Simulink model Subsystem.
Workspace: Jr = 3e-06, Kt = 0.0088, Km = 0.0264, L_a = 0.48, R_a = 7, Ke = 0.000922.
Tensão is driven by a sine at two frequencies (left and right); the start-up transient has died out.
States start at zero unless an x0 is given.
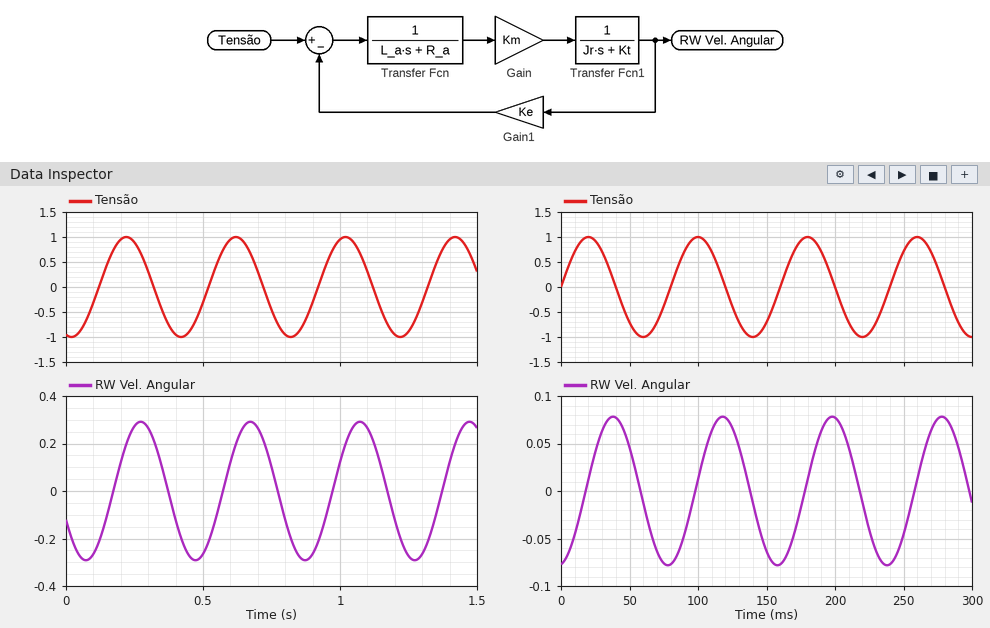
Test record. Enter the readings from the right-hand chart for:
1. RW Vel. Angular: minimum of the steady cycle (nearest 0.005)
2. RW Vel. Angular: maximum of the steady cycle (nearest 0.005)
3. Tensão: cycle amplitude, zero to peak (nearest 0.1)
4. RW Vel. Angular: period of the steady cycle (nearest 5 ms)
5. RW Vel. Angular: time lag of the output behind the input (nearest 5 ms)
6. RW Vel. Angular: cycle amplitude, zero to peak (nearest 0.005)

-0.080
0.080
1.0
80 ms
20 ms
0.080
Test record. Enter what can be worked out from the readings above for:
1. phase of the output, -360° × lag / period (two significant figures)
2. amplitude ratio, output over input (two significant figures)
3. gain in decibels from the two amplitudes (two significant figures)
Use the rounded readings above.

-90°
0.080
-22 dB
